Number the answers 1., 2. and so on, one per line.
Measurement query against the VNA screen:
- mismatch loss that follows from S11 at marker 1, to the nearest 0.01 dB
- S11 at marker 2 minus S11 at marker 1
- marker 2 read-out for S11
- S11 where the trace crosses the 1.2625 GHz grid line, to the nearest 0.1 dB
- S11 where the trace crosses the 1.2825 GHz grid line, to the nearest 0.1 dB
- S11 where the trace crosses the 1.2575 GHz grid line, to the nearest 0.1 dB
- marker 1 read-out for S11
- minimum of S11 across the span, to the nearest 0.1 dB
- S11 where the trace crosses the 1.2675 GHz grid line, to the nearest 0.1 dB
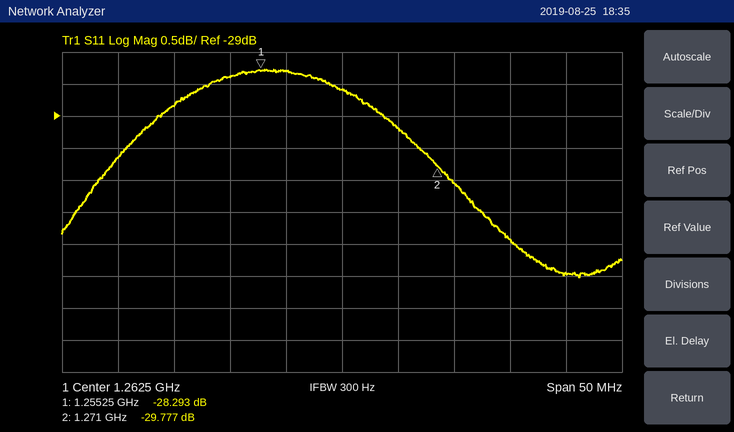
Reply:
1. 0.01 dB
2. -1.484 dB
3. -29.777 dB
4. -28.6 dB
5. -31.5 dB
6. -28.3 dB
7. -28.293 dB
8. -31.5 dB
9. -29.2 dB
